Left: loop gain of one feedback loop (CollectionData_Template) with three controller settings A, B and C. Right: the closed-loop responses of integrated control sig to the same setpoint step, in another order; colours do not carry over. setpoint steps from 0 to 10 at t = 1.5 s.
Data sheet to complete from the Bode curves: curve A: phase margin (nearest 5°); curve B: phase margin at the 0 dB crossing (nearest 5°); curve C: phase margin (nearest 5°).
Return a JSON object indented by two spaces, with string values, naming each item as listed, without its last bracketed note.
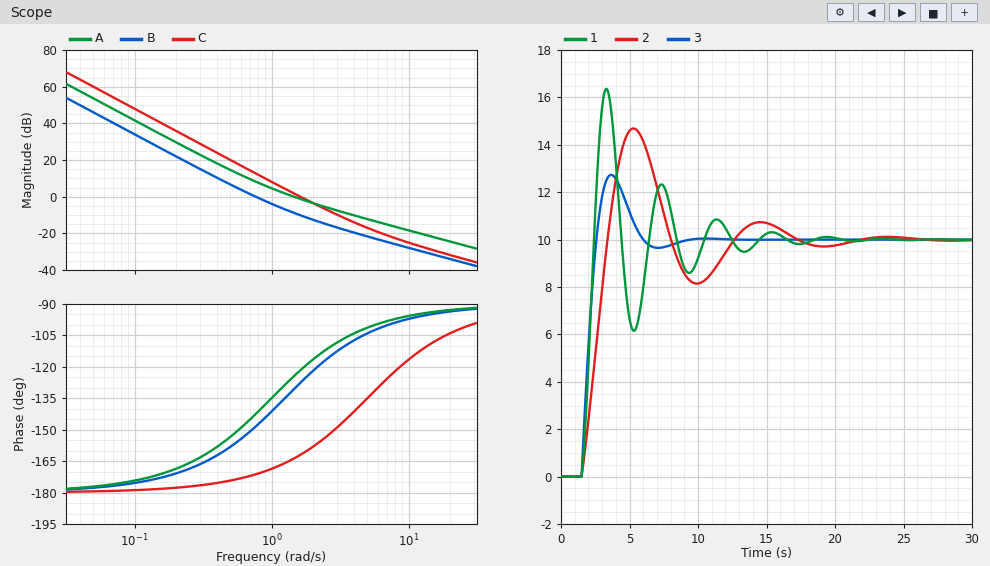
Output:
{
  "curve A: phase margin": "55°",
  "curve B: phase margin at the 0 dB crossing": "30°",
  "curve C: phase margin": "20°"
}
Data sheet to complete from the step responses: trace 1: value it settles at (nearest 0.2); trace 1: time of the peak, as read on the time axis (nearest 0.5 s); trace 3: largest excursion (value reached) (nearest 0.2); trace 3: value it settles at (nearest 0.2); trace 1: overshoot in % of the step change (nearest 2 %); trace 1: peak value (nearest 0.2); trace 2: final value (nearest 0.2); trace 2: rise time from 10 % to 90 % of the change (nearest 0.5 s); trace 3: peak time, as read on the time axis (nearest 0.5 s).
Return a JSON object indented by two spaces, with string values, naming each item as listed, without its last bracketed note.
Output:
{
  "trace 1: value it settles at": "10.0",
  "trace 1: time of the peak, as read on the time axis": "3.5 s",
  "trace 3: largest excursion (value reached)": "12.8",
  "trace 3: value it settles at": "10.0",
  "trace 1: overshoot in % of the step change": "64 %",
  "trace 1: peak value": "16.4",
  "trace 2: final value": "10.0",
  "trace 2: rise time from 10 % to 90 % of the change": "1.5 s",
  "trace 3: peak time, as read on the time axis": "3.5 s"
}
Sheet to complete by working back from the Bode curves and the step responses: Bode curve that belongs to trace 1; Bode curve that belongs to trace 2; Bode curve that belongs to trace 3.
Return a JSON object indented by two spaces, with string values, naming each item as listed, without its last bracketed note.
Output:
{
  "Bode curve that belongs to trace 1": "C",
  "Bode curve that belongs to trace 2": "B",
  "Bode curve that belongs to trace 3": "A"
}
